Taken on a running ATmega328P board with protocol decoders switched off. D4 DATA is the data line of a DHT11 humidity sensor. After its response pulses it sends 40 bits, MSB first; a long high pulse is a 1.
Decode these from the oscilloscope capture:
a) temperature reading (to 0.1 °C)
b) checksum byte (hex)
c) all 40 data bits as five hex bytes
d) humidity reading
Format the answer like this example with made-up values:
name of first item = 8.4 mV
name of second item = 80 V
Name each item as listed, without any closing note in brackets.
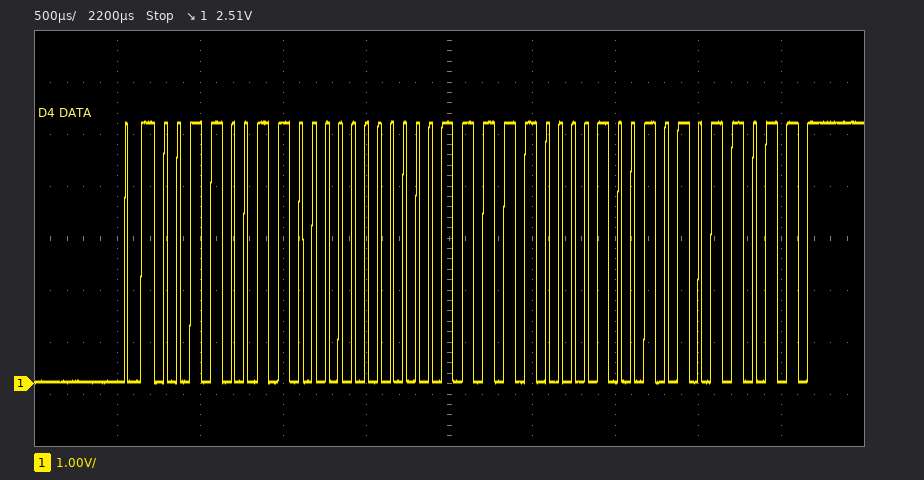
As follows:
temperature reading = 31.9 °C
checksum byte = 0x5B
all 40 data bits as five hex bytes = 33 00 1F 09 5B
humidity reading = 51 %
